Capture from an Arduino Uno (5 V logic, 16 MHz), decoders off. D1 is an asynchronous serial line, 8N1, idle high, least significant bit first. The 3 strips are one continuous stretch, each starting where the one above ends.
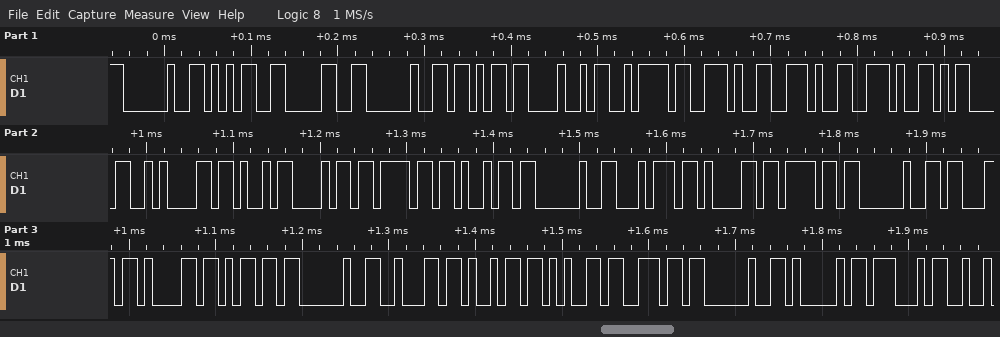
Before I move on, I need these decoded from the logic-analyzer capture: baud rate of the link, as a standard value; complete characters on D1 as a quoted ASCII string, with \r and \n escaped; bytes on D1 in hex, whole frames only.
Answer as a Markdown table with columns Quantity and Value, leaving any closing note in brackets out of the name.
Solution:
| Quantity | Value |
|---|---|
| baud rate of the link, as a standard value | 115200 baud |
| complete characters on D1 as a quoted ASCII string, with \r and \n escaped | " 50 kHz...\r\nKhoi tao cam bien AG" |
| bytes on D1 in hex, whole frames only | 0x20 0x35 0x30 0x20 0x6B 0x48 0x7A 0x2E 0x2E 0x2E 0x0D 0x0A 0x4B 0x68 0x6F 0x69 0x20 0x74 0x61 0x6F 0x20 0x63 0x61 0x6D 0x20 0x62 0x69 0x65 0x6E 0x20 0x41 0x47 |
